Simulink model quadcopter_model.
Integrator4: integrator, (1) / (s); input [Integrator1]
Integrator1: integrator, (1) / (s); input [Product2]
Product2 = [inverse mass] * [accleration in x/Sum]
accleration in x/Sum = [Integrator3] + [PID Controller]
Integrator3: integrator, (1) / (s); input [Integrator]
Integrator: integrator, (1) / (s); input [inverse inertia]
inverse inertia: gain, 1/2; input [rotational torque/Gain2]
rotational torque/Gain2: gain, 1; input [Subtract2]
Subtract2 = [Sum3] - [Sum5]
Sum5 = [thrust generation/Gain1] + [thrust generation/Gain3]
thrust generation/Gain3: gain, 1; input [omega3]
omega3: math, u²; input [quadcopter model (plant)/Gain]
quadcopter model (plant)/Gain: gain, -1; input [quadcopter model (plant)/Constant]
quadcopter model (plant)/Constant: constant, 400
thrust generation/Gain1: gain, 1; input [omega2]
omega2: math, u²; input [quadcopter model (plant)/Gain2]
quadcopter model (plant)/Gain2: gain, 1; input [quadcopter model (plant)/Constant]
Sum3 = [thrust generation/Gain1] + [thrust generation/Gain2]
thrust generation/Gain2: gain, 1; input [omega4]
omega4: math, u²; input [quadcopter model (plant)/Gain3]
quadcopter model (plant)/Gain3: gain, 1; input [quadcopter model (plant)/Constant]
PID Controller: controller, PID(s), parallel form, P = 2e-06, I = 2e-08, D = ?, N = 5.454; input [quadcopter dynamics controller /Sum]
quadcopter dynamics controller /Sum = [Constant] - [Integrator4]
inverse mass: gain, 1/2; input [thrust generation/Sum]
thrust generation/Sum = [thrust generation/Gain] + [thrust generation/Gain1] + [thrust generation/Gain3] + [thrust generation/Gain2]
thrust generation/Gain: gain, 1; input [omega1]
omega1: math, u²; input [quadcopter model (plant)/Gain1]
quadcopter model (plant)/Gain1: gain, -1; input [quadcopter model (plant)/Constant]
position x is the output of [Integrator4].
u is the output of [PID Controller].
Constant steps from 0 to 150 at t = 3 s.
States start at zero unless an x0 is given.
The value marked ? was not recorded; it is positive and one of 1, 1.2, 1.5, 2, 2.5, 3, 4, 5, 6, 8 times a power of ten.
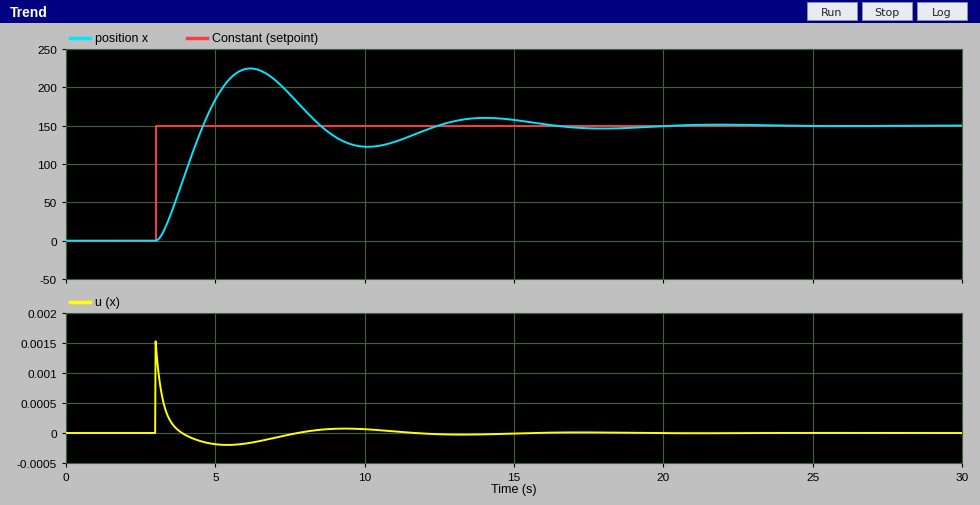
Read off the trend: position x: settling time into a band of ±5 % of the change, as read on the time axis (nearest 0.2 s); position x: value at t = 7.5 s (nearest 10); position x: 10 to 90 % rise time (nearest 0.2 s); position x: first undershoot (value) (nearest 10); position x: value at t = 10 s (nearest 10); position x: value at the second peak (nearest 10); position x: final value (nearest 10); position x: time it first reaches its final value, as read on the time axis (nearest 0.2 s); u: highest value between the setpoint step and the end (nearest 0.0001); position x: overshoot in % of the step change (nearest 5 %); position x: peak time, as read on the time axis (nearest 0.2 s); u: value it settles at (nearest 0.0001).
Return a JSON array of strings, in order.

["15.0 s", "190", "1.2 s", "120", "120", "160", "150", "4.6 s", "0.0015", "50 %", "6.2 s", "0.0000"]
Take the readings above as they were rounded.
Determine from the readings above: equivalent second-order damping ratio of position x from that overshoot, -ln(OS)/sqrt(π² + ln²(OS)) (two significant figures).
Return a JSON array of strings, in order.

["0.22"]
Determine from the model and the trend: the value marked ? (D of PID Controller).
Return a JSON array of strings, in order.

["1.5e-06"]
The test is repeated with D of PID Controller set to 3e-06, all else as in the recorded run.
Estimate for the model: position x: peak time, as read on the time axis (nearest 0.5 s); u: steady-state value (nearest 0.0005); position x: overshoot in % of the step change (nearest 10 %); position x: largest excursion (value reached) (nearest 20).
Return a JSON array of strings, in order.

["5.5 s", "0.0000", "30 %", "200"]
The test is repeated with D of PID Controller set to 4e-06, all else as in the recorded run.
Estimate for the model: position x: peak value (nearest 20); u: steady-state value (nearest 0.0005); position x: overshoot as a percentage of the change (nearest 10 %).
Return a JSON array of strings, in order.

["180", "0.0000", "20 %"]
